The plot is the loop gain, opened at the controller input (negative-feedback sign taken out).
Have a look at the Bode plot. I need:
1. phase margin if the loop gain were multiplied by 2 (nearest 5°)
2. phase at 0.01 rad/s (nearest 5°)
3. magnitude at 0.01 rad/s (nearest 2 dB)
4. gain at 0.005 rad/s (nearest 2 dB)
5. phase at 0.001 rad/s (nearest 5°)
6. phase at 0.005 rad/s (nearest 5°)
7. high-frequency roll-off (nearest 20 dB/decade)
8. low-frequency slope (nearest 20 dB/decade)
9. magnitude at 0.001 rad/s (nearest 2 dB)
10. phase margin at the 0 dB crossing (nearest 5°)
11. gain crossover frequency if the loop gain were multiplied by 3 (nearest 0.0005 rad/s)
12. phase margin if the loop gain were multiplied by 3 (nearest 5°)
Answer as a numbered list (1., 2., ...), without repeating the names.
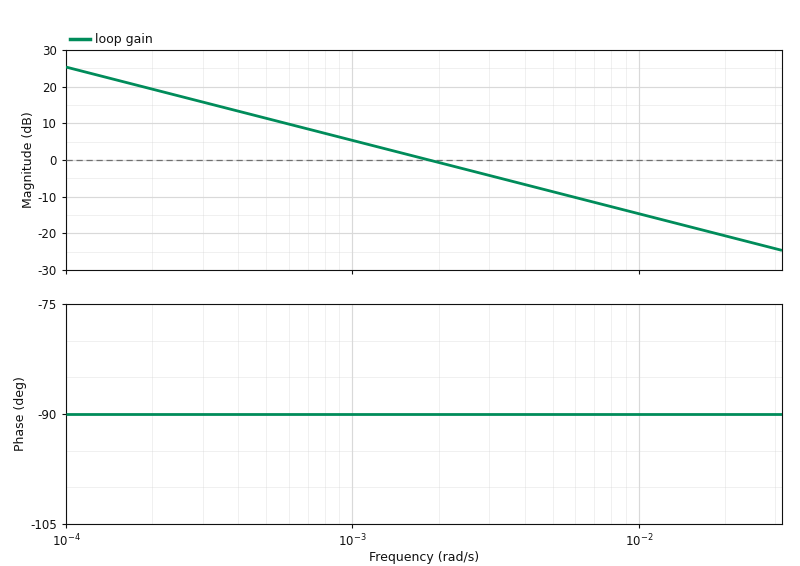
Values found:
1. 90°
2. -90°
3. -14 dB
4. -8 dB
5. -90°
6. -90°
7. -20 dB/decade
8. -20 dB/decade
9. 6 dB
10. 90°
11. 0.0055 rad/s
12. 90°
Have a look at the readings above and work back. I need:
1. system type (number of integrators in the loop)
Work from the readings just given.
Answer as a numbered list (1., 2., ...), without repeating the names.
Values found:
1. 1
